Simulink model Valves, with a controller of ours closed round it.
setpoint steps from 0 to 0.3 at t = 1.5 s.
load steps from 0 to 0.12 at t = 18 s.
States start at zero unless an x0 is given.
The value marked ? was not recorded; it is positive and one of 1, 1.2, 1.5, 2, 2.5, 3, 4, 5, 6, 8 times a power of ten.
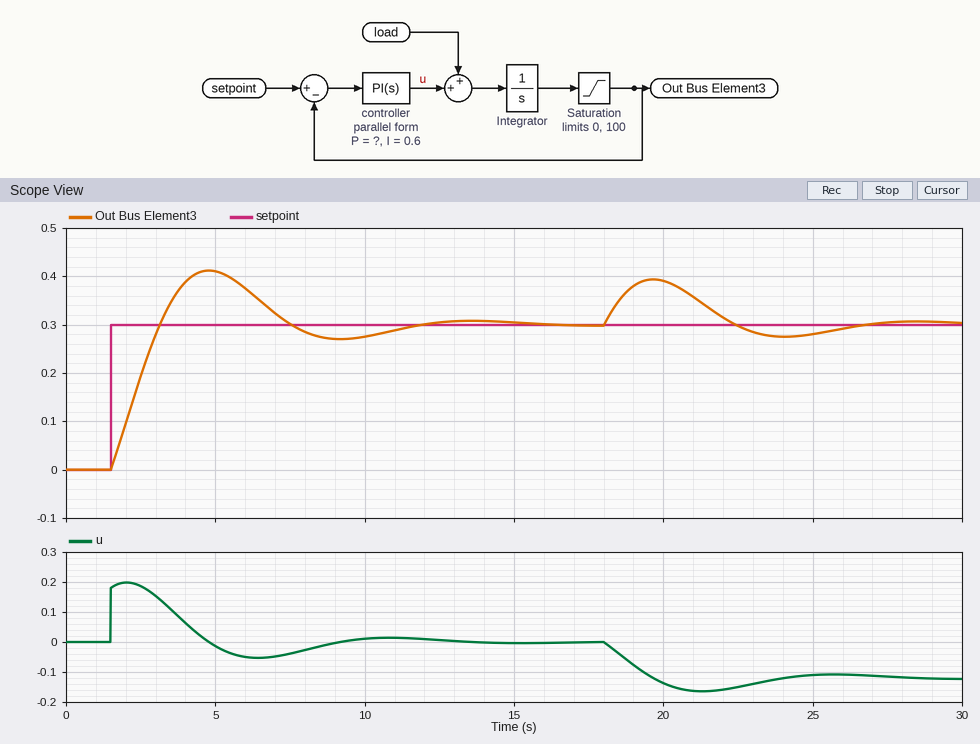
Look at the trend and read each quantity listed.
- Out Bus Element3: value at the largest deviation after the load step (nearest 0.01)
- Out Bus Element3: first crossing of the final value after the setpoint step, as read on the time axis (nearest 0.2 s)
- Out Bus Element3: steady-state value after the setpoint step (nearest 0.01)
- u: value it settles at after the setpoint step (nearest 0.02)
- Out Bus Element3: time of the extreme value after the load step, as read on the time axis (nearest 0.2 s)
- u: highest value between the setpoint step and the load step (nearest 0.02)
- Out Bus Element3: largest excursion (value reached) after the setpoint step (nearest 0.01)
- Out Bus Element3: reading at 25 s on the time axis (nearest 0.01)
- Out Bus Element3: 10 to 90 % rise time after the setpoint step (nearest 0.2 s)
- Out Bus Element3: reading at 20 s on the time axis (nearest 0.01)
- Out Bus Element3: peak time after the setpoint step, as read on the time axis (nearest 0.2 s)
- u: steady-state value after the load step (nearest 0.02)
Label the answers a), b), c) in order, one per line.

a) 0.39
b) 3.2 s
c) 0.30
d) 0.00
e) 19.6 s
f) 0.20
g) 0.41
h) 0.28
i) 1.2 s
j) 0.39
k) 4.8 s
l) -0.12
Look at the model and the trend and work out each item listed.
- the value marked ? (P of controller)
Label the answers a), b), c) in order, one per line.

a) 0.6
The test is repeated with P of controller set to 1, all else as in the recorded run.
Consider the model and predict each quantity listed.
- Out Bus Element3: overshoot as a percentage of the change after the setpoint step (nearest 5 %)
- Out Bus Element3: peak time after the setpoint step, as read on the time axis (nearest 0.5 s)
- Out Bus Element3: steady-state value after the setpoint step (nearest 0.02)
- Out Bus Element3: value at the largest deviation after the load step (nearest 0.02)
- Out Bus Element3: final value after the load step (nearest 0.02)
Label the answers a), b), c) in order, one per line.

a) 25 %
b) 4.5 s
c) 0.30
d) 0.38
e) 0.30
